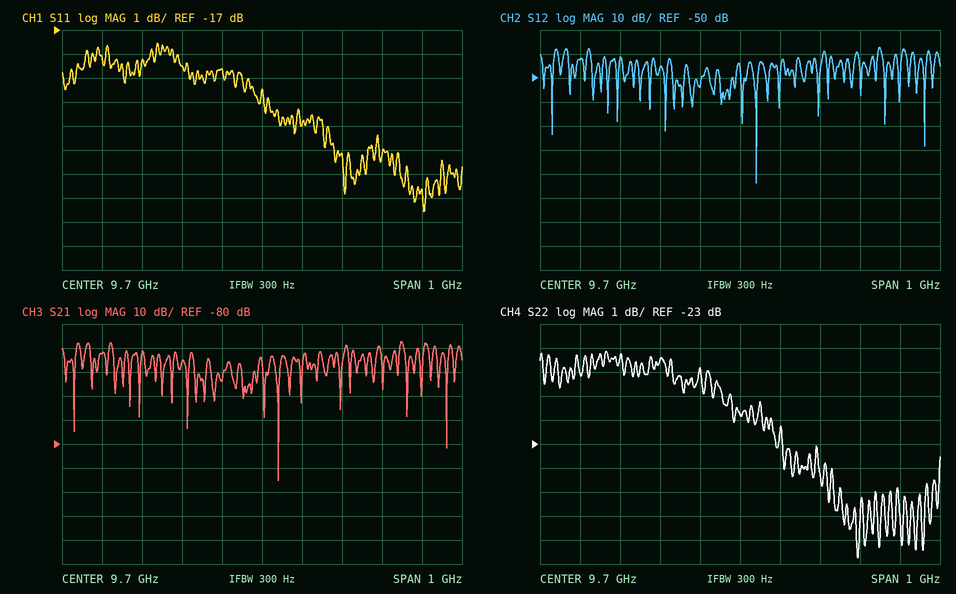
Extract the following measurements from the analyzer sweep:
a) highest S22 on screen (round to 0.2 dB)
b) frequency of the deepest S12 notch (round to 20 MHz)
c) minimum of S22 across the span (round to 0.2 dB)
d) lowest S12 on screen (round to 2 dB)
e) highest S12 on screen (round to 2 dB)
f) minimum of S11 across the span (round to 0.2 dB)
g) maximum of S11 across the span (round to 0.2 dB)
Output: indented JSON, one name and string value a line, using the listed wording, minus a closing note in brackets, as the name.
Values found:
{
  "highest S22 on screen": "-19.2 dB",
  "frequency of the deepest S12 notch": "9.74 GHz",
  "minimum of S22 across the span": "-27.8 dB",
  "lowest S12 on screen": "-94 dB",
  "highest S12 on screen": "-38 dB",
  "minimum of S11 across the span": "-24.6 dB",
  "maximum of S11 across the span": "-17.6 dB"
}
